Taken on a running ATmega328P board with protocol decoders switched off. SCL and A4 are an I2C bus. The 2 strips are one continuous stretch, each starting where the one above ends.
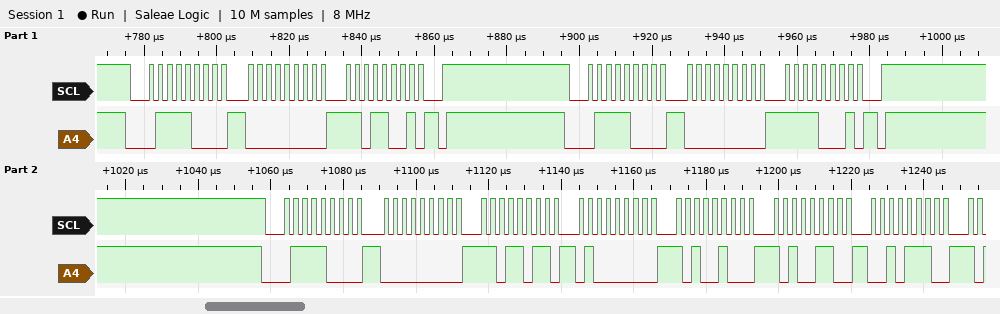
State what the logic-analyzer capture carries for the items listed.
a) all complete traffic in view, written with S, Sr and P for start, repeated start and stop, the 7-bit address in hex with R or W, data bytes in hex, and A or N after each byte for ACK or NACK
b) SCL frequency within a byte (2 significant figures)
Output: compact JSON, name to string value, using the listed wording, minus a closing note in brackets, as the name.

{"all complete traffic in view, written with S, Sr and P for start, repeated start and stop, the 7-bit address in hex with R or W, data bytes in hex, and A or N after each byte for ACK or NACK": "S 3CW A 00 A D9 A P S 3CW A 00 A F1 A P S 3CW A 00 A DB A 40 A A4 A A6 A 2E A", "SCL frequency within a byte": "400 kHz"}
